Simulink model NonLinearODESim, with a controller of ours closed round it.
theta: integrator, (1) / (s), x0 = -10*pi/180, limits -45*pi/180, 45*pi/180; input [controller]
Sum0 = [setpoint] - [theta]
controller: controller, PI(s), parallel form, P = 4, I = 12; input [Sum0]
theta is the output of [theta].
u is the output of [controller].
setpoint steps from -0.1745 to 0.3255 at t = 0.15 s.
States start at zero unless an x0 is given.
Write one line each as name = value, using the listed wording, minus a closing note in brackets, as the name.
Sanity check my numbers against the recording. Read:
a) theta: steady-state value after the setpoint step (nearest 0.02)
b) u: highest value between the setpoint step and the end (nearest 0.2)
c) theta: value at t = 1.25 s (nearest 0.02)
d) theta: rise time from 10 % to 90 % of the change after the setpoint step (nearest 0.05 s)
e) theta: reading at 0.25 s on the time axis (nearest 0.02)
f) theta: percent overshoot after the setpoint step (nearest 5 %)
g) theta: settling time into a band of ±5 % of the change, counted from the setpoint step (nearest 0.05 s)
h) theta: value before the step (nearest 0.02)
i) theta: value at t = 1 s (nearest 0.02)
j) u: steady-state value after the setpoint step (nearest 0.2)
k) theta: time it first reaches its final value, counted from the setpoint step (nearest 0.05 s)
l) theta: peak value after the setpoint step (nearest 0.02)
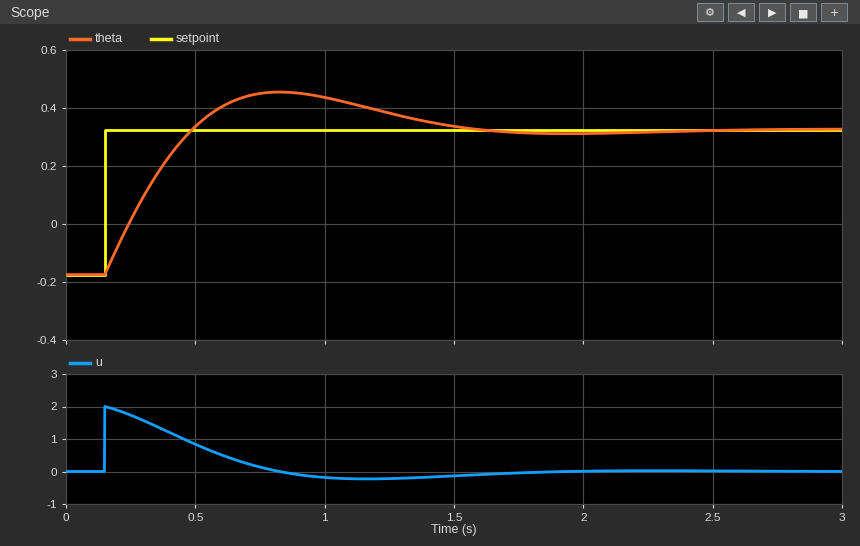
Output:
theta: steady-state value after the setpoint step = 0.32
u: highest value between the setpoint step and the end = 2.0
theta: value at t = 1.25 s = 0.38
theta: rise time from 10 % to 90 % of the change after the setpoint step = 0.25 s
theta: reading at 0.25 s on the time axis = 0.02
theta: percent overshoot after the setpoint step = 25 %
theta: settling time into a band of ±5 % of the change, counted from the setpoint step = 1.25 s
theta: value before the step = -0.18
theta: value at t = 1 s = 0.44
u: steady-state value after the setpoint step = 0.0
theta: time it first reaches its final value, counted from the setpoint step = 0.35 s
theta: peak value after the setpoint step = 0.46
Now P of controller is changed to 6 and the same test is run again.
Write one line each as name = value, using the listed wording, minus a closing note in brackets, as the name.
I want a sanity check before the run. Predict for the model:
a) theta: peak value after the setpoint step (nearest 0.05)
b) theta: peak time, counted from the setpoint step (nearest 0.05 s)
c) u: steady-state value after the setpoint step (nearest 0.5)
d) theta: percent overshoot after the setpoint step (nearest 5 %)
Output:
theta: peak value after the setpoint step = 0.40
theta: peak time, counted from the setpoint step = 0.60 s
u: steady-state value after the setpoint step = 0.0
theta: percent overshoot after the setpoint step = 15 %
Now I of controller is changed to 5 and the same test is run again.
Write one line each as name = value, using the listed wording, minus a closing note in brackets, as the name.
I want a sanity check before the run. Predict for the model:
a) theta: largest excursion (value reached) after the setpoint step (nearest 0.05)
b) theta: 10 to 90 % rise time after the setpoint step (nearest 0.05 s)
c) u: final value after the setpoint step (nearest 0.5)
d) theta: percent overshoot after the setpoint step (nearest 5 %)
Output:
theta: largest excursion (value reached) after the setpoint step = 0.40
theta: 10 to 90 % rise time after the setpoint step = 0.35 s
u: final value after the setpoint step = 0.0
theta: percent overshoot after the setpoint step = 15 %
